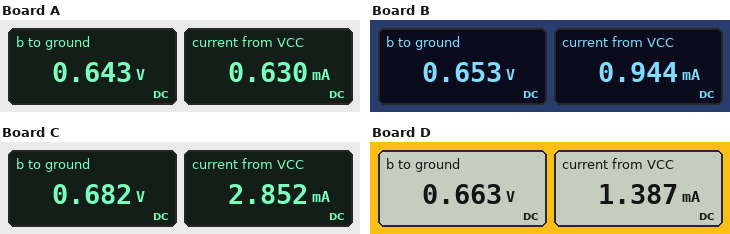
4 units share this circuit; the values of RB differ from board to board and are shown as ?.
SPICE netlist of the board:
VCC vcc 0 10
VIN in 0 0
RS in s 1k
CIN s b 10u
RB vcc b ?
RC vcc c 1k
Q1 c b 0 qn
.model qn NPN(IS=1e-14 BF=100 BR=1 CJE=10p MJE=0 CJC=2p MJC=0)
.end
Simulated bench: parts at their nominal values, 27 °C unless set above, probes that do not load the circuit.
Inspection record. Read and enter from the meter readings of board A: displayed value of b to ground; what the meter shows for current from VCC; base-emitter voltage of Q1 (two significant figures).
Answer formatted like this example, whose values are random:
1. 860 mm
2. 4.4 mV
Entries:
1. 0.643 V
2. 0.630 mA
3. 640 mV
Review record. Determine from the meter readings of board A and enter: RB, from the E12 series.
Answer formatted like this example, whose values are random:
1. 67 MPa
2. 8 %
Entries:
1. 1.5 MΩ
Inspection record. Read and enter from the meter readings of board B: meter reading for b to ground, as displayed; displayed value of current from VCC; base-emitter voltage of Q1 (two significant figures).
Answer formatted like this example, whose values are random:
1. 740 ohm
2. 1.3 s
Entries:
1. 0.653 V
2. 0.944 mA
3. 650 mV
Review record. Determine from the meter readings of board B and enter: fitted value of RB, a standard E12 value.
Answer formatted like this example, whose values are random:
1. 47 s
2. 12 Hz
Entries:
1. 1 MΩ
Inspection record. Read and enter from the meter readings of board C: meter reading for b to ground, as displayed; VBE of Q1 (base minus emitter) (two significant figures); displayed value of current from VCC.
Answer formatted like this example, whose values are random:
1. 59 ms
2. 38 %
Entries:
1. 0.682 V
2. 680 mV
3. 2.852 mA
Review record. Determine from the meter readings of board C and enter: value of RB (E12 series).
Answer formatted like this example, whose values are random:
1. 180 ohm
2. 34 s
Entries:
1. 330 kΩ
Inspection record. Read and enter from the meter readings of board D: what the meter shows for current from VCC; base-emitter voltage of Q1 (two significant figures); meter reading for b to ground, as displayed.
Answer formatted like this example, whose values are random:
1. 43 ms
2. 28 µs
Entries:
1. 1.387 mA
2. 660 mV
3. 0.663 V
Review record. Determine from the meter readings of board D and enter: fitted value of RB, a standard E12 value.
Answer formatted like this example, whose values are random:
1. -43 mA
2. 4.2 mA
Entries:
1. 680 kΩ
